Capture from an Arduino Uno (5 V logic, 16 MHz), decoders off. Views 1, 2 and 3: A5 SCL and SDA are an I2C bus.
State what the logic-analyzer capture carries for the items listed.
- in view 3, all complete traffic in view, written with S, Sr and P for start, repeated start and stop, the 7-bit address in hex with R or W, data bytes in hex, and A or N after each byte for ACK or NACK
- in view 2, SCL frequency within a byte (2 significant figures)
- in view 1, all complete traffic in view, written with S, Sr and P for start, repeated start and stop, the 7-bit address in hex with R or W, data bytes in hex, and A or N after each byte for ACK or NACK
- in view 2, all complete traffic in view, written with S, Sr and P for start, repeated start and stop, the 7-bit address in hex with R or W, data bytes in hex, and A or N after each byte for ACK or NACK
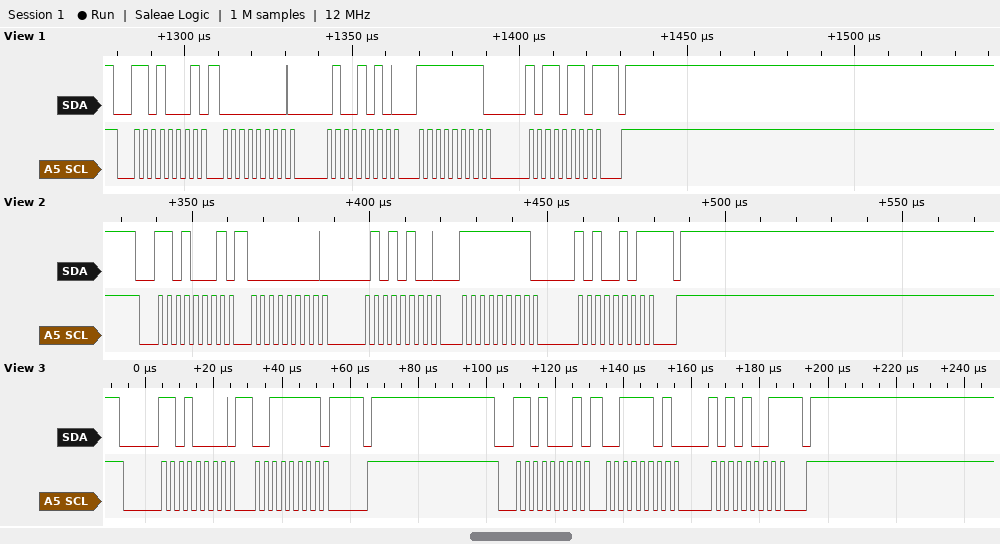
S 68W A 3F A P S 68R A 3D A A9 N P
400 kHz
S 68R A 00 A 4A A FF A B6 N P
S 68R A 00 A 54 A FF A A5 N P
